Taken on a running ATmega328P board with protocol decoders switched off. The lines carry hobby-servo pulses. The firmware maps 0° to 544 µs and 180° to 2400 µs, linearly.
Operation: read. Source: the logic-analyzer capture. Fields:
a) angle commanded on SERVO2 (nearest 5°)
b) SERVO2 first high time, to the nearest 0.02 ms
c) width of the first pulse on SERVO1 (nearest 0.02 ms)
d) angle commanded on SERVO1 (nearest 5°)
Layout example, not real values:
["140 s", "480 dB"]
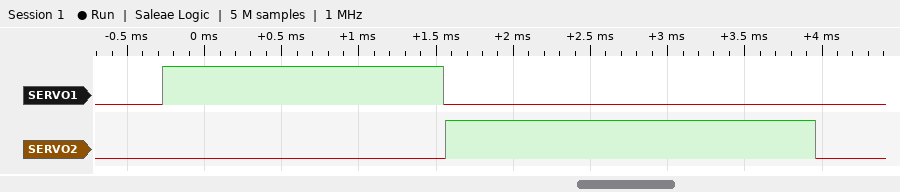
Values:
["180°", "2.40 ms", "1.82 ms", "125°"]
